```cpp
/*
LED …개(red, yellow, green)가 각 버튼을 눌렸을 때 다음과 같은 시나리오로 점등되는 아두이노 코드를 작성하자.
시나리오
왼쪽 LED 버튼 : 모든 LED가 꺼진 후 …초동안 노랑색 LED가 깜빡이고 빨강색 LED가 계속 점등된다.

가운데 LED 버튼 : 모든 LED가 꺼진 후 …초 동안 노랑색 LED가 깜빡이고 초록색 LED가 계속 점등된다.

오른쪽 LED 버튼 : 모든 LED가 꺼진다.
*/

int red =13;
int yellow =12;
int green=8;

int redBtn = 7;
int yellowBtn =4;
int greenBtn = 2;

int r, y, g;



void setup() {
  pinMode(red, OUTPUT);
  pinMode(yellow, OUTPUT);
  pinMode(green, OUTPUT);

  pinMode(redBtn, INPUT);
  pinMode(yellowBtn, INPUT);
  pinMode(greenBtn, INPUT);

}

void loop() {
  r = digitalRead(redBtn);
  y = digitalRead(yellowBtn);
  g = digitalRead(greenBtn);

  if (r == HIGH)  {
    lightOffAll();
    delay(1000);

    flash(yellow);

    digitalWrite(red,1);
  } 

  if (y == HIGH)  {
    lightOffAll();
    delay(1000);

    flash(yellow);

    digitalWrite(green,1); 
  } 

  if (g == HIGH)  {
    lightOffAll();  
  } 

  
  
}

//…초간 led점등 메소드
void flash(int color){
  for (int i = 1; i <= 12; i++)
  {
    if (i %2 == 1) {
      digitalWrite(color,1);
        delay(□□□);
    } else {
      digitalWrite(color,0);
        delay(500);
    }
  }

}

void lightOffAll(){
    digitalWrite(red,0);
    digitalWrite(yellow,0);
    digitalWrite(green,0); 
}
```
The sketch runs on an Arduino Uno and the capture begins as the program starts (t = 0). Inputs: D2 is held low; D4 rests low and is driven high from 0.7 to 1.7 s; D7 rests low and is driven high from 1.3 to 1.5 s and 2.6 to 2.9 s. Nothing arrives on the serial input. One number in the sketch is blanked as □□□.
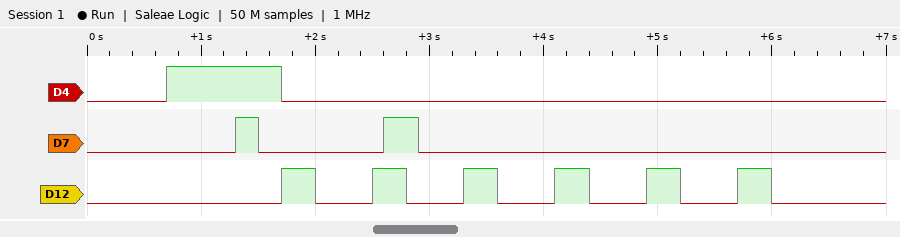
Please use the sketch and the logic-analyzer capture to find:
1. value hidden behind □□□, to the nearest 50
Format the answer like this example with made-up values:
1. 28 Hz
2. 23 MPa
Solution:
1. 300
